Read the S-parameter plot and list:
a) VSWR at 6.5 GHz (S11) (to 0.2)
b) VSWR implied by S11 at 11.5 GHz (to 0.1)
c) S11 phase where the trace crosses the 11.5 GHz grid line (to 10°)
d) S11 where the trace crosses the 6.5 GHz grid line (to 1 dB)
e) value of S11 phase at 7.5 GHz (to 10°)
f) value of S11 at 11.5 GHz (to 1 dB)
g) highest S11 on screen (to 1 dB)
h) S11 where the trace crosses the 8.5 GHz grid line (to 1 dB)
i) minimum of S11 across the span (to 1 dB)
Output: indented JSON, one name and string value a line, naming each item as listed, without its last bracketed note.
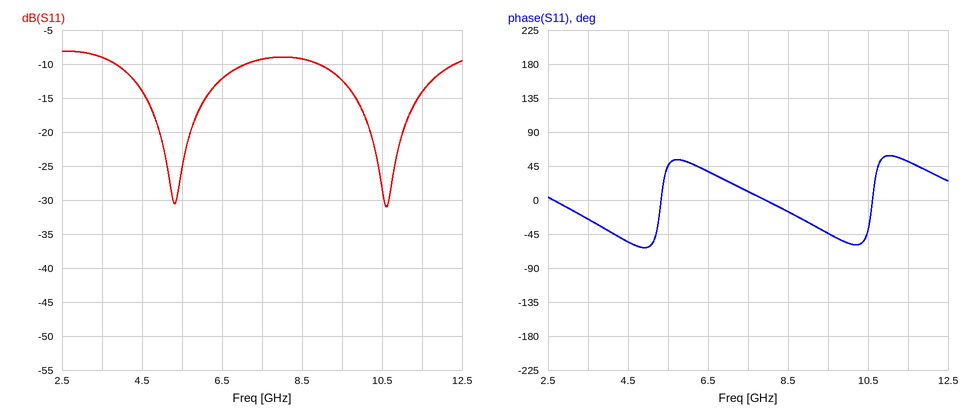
{
  "VSWR at 6.5 GHz (S11)": "1.6",
  "VSWR implied by S11 at 11.5 GHz": "1.5",
  "S11 phase where the trace crosses the 11.5 GHz grid line": "50°",
  "S11 where the trace crosses the 6.5 GHz grid line": "-12 dB",
  "value of S11 phase at 7.5 GHz": "10°",
  "value of S11 at 11.5 GHz": "-14 dB",
  "highest S11 on screen": "-8 dB",
  "S11 where the trace crosses the 8.5 GHz grid line": "-9 dB",
  "minimum of S11 across the span": "-31 dB"
}
